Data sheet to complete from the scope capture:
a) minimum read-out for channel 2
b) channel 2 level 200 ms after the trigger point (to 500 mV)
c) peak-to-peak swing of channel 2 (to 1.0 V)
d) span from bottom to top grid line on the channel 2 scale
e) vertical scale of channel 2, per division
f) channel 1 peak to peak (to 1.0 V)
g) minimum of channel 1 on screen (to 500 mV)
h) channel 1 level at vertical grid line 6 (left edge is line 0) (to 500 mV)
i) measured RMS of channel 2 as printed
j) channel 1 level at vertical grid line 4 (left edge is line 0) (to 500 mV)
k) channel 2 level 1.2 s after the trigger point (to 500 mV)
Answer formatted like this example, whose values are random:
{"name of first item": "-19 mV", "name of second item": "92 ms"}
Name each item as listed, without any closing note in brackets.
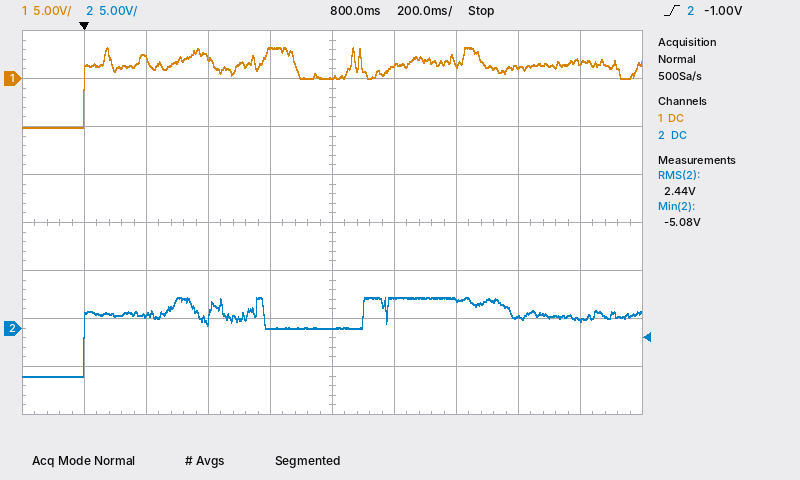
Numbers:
{"minimum read-out for channel 2": "-5.08 V", "channel 2 level 200 ms after the trigger point": "1.5 V", "peak-to-peak swing of channel 2": "8.0 V", "span from bottom to top grid line on the channel 2 scale": "40 V", "vertical scale of channel 2, per division": "5 V", "channel 1 peak to peak": "8.0 V", "minimum of channel 1 on screen": "-5.0 V", "channel 1 level at vertical grid line 6 (left edge is line 0)": "1.5 V", "measured RMS of channel 2 as printed": "2.44 V", "channel 1 level at vertical grid line 4 (left edge is line 0)": "3.0 V", "channel 2 level 1.2 s after the trigger point": "3.0 V"}
